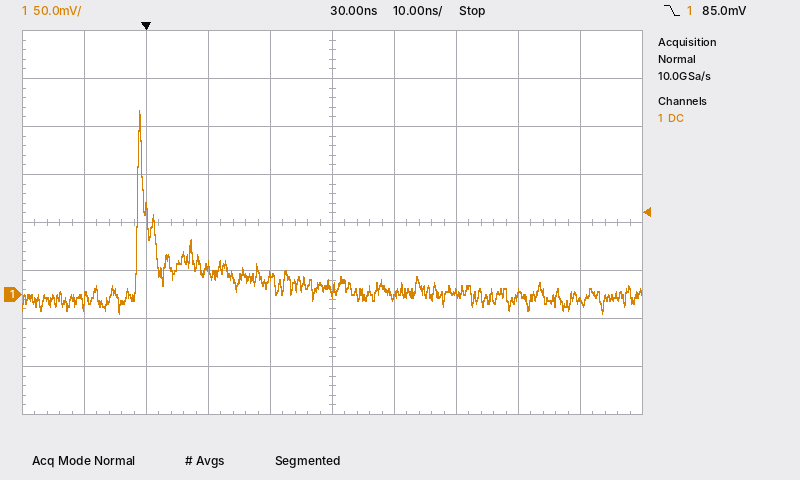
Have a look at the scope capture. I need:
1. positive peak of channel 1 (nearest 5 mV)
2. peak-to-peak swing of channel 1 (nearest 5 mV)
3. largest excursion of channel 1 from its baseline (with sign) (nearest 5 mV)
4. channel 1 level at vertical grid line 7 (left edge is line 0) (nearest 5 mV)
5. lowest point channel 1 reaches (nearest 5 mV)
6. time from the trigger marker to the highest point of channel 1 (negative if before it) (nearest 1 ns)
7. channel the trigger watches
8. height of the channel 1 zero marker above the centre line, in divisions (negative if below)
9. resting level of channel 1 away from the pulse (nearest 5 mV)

190 mV
210 mV
+190 mV
0 mV
-20 mV
-1 ns
channel 1
-1.5 div
0 mV
